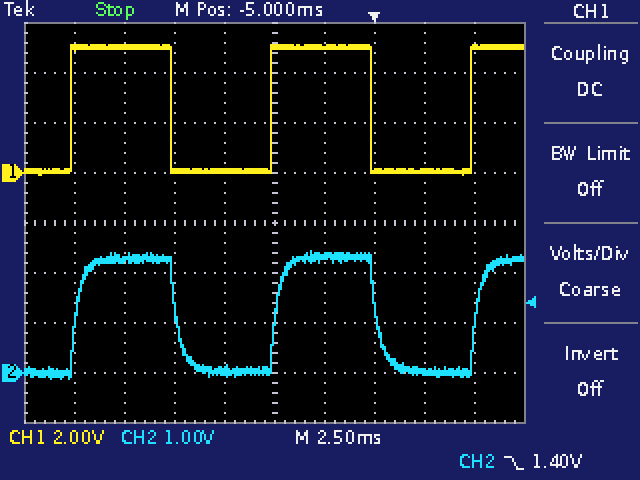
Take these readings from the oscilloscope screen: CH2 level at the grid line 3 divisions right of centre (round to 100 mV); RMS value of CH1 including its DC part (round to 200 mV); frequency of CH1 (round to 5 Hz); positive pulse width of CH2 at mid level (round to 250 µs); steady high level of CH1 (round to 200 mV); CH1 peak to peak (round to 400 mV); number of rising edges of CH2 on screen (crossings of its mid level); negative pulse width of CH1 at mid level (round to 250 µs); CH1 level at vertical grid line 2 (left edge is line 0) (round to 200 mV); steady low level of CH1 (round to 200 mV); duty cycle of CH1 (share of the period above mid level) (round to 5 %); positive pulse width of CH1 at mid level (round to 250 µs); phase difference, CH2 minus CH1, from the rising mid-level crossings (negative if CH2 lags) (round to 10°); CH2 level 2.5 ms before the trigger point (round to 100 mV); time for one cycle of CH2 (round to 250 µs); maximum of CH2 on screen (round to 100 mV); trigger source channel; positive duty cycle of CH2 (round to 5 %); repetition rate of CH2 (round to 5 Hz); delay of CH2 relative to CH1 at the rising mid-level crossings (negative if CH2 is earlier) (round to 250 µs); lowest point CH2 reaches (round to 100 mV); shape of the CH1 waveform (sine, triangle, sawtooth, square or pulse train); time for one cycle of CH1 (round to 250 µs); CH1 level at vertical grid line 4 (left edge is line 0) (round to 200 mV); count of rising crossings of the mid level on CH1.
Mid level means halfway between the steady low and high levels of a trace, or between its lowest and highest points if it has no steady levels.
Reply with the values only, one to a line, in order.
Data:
0.0 V
3.6 V
100 Hz
5.00 ms
5.0 V
5.2 V
3
5.00 ms
5.0 V
0.0 V
50 %
5.00 ms
-10°
2.3 V
10.00 ms
2.4 V
CH2
50 %
100 Hz
+250 µs
-100 mV
square
10.00 ms
0.0 V
3
